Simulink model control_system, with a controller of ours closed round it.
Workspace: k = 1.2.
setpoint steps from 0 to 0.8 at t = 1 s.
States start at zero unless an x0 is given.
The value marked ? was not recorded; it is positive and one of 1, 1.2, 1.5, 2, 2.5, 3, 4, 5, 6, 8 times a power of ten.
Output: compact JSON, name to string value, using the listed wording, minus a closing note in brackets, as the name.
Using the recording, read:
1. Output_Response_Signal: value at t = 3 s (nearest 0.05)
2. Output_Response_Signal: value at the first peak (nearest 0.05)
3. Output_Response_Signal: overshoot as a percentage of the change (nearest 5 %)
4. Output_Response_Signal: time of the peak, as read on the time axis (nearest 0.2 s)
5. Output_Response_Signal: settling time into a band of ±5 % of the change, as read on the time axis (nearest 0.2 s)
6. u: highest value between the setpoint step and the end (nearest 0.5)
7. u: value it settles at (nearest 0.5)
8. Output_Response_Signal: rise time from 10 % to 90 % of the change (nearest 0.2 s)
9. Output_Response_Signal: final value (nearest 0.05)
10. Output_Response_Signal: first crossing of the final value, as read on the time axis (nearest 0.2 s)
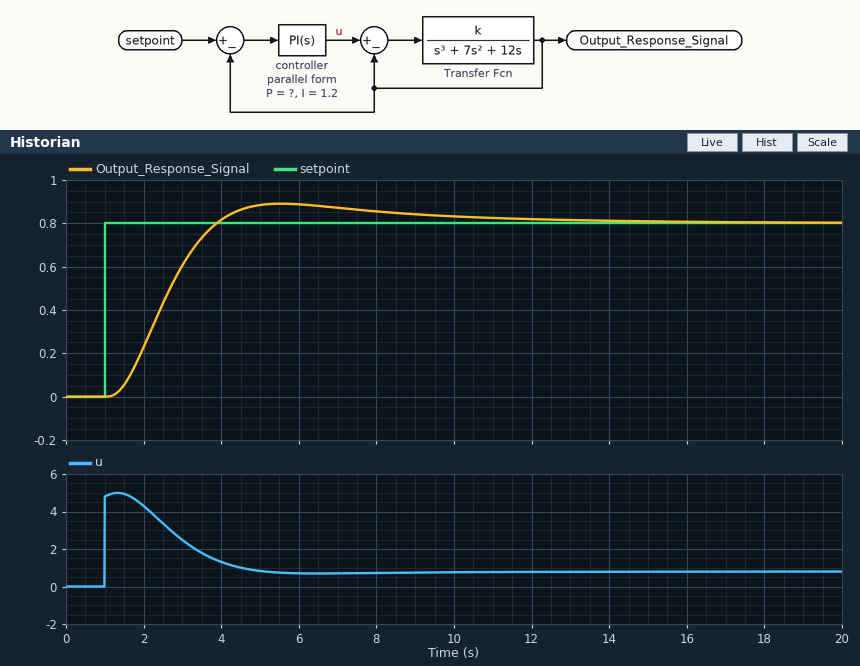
{"Output_Response_Signal: value at t = 3 s": "0.60", "Output_Response_Signal: value at the first peak": "0.90", "Output_Response_Signal: overshoot as a percentage of the change": "10 %", "Output_Response_Signal: time of the peak, as read on the time axis": "5.6 s", "Output_Response_Signal: settling time into a band of ±5 % of the change, as read on the time axis": "9.2 s", "u: highest value between the setpoint step and the end": "5.0", "u: value it settles at": "1.0", "Output_Response_Signal: rise time from 10 % to 90 % of the change": "1.8 s", "Output_Response_Signal: final value": "0.80", "Output_Response_Signal: first crossing of the final value, as read on the time axis": "3.8 s"}
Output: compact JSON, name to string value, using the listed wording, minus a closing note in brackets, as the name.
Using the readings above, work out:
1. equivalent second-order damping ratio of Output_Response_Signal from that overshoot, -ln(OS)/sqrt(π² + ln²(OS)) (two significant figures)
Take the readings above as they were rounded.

{"equivalent second-order damping ratio of Output_Response_Signal from that overshoot, -ln(OS)/sqrt(π² + ln²(OS))": "0.59"}
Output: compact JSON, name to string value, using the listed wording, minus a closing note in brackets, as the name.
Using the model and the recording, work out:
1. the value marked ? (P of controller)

{"the value marked ?": "6"}
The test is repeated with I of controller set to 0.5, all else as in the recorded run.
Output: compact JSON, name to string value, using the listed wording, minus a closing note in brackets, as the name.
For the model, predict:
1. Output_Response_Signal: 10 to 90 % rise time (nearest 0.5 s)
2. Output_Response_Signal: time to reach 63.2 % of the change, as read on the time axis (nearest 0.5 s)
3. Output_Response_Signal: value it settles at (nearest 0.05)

{"Output_Response_Signal: 10 to 90 % rise time": "2.5 s", "Output_Response_Signal: time to reach 63.2 % of the change, as read on the time axis": "3.0 s", "Output_Response_Signal: value it settles at": "0.80"}
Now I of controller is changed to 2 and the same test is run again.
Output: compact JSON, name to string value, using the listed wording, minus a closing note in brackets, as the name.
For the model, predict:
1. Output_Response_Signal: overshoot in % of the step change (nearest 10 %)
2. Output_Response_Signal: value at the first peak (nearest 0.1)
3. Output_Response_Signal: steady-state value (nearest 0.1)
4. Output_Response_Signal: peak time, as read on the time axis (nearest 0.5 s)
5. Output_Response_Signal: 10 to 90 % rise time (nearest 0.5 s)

{"Output_Response_Signal: overshoot in % of the step change": "20 %", "Output_Response_Signal: value at the first peak": "1.0", "Output_Response_Signal: steady-state value": "0.8", "Output_Response_Signal: peak time, as read on the time axis": "5.0 s", "Output_Response_Signal: 10 to 90 % rise time": "1.5 s"}
